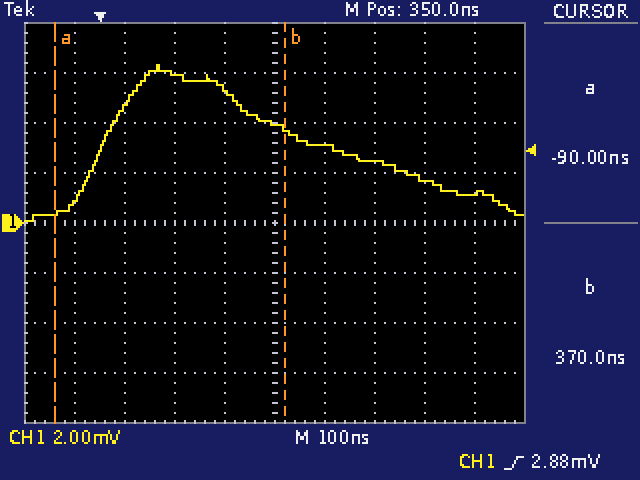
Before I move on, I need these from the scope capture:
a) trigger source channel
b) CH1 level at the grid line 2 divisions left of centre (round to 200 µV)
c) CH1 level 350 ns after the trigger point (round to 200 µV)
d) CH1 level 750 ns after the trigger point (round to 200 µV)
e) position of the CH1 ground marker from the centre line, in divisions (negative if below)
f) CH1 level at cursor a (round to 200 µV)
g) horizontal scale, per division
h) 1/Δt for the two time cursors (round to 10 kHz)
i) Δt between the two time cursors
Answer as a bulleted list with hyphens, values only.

- CH1
- 6.0 mV
- 4.0 mV
- 1.2 mV
- 0.0 div
- 400 µV
- 100 ns
- 2.17 MHz
- 460 ns
